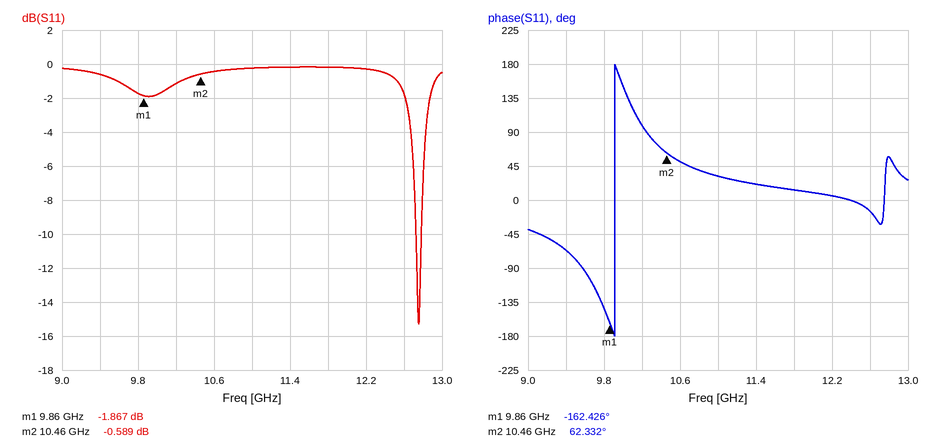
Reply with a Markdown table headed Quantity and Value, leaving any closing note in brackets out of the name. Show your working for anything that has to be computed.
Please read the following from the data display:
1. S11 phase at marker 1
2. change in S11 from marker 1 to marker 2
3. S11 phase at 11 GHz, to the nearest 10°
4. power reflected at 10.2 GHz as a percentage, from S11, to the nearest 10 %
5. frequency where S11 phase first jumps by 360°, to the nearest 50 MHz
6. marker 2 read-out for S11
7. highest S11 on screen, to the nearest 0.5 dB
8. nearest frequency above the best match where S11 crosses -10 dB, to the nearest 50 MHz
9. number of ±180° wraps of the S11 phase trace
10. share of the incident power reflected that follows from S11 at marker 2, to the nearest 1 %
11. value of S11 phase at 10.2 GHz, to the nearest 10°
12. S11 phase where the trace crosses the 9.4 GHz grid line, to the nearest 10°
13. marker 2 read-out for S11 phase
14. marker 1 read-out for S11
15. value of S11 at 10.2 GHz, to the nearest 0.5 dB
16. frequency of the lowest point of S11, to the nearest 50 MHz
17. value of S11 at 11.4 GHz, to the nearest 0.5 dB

| Quantity | Value |
|---|---|
| S11 phase at marker 1 | -162.426° |
| change in S11 from marker 1 to marker 2 | -0.589 − (-1.867) = 1.278 dB |
| S11 phase at 11 GHz, to the nearest 10° | 30° |
| power reflected at 10.2 GHz as a percentage, from S11, to the nearest 10 % | 10^(-1/10) ≈ 79.4 %, so 80 % to the nearest 10 % |
| frequency where S11 phase first jumps by 360°, to the nearest 50 MHz | 9.90 GHz |
| marker 2 read-out for S11 | -0.589 dB |
| highest S11 on screen, to the nearest 0.5 dB | 0.0 dB |
| nearest frequency above the best match where S11 crosses -10 dB, to the nearest 50 MHz | 12.80 GHz |
| number of ±180° wraps of the S11 phase trace | 1 |
| share of the incident power reflected that follows from S11 at marker 2, to the nearest 1 % | 10^(-0.589/10) ≈ 87 % |
| value of S11 phase at 10.2 GHz, to the nearest 10° | 100° |
| S11 phase where the trace crosses the 9.4 GHz grid line, to the nearest 10° | -70° |
| marker 2 read-out for S11 phase | 62.332° |
| marker 1 read-out for S11 | -1.867 dB |
| value of S11 at 10.2 GHz, to the nearest 0.5 dB | -1.0 dB |
| frequency of the lowest point of S11, to the nearest 50 MHz | 12.75 GHz |
| value of S11 at 11.4 GHz, to the nearest 0.5 dB | 0.0 dB |
